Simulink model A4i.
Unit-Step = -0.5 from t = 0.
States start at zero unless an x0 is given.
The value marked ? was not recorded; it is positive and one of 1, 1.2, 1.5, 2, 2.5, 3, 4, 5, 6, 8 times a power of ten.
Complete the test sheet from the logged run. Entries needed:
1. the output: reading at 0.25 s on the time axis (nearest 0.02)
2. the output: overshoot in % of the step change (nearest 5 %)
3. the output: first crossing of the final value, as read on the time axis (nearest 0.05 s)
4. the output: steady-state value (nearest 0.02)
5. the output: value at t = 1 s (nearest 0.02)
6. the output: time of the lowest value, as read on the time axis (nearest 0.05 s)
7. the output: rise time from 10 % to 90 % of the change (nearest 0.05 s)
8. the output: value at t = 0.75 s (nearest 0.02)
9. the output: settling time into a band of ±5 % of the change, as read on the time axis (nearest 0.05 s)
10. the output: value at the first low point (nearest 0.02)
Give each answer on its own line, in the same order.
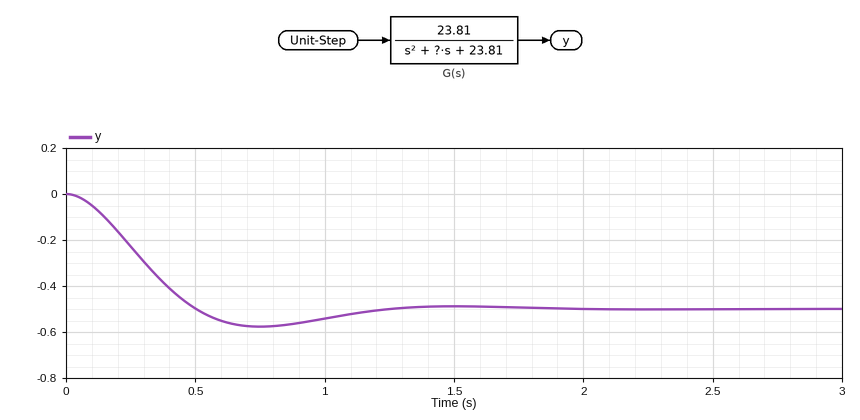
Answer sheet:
-0.22
15 %
0.50 s
-0.50
-0.54
0.75 s
0.35 s
-0.58
1.10 s
-0.58
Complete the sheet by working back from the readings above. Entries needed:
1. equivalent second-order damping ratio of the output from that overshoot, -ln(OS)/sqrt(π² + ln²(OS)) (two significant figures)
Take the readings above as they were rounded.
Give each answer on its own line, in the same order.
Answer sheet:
0.52
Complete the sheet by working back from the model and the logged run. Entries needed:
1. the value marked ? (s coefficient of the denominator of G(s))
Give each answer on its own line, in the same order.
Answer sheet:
5
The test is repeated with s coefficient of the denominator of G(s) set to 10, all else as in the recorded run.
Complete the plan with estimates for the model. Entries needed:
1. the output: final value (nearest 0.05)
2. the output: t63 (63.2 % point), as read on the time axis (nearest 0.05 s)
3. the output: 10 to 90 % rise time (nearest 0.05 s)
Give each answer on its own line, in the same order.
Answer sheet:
-0.50
0.45 s
0.70 s
